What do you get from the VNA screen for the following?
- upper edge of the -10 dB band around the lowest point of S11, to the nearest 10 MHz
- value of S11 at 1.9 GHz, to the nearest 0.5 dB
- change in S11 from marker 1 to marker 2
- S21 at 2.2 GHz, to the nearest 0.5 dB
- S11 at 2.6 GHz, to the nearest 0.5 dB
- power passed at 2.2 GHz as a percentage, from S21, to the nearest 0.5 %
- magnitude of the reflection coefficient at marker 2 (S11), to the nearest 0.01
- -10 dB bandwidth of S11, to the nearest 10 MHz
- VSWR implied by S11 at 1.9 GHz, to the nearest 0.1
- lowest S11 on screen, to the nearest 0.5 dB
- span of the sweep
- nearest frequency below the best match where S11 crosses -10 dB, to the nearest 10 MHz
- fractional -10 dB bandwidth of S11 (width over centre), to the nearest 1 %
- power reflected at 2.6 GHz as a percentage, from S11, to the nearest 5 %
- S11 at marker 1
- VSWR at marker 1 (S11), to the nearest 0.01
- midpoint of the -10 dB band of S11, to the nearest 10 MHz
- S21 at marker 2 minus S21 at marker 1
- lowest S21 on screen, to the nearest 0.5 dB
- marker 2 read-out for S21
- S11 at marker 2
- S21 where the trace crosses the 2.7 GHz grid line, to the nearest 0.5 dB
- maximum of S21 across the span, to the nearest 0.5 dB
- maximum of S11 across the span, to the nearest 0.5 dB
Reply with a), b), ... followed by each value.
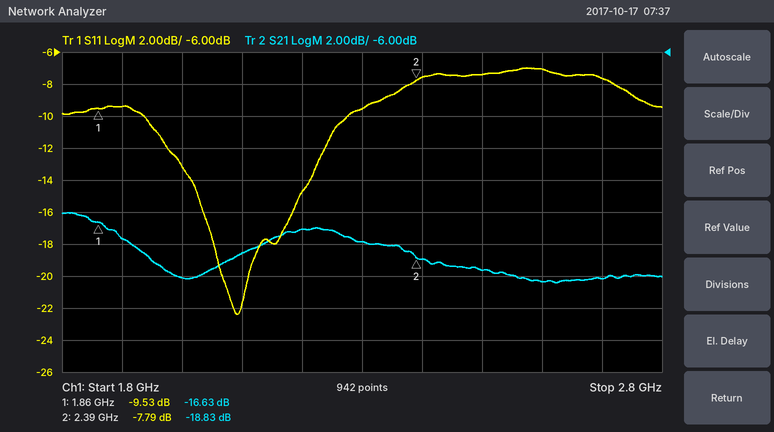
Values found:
a) 2.28 GHz
b) -9.5 dB
c) 1.74 dB
d) -17.0 dB
e) -7.0 dB
f) 2.0 %
g) 0.41
h) 340 MHz
i) 2.0
j) -22.5 dB
k) 1 GHz
l) 1.94 GHz
m) 16 %
n) 20 %
o) -9.53 dB
p) 2.00
q) 2.11 GHz
r) -2.20 dB
s) -20.5 dB
t) -18.83 dB
u) -7.79 dB
v) -20.0 dB
w) -16.0 dB
x) -7.0 dB
